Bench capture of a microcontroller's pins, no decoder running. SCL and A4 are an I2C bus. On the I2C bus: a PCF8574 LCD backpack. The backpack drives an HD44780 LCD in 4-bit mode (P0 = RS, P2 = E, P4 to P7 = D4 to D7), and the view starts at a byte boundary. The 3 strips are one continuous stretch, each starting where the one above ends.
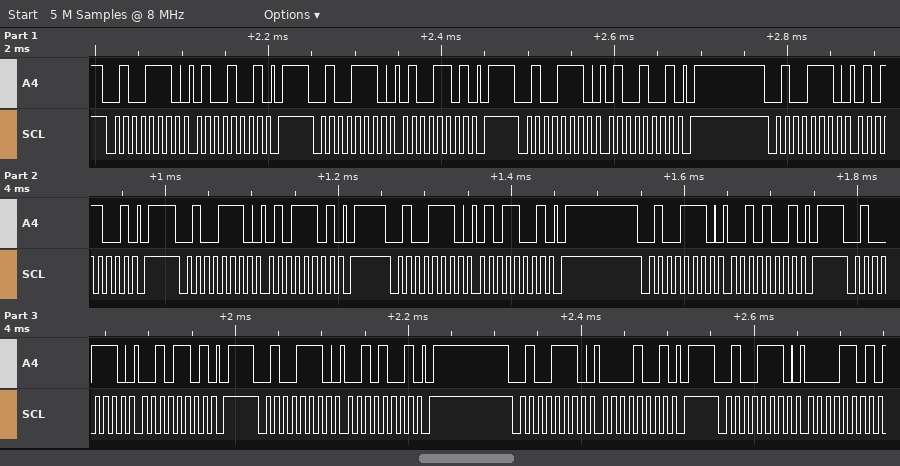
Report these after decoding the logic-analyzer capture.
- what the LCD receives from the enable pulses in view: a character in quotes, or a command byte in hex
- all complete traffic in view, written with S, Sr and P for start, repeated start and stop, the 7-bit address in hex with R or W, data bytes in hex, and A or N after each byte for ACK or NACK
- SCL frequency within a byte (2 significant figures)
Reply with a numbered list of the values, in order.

1. 'E'
2. S 27W A 49 A P S 27W A 4D A P S 27W A 49 A P S 27W A 59 A P S 27W A 5D A P S 27W A 59 A P S 27W A 29 A P S 27W A 2D A P S 27W A 29 A P S 27W A 09 A P S 27W A 0D A
3. 100 kHz
